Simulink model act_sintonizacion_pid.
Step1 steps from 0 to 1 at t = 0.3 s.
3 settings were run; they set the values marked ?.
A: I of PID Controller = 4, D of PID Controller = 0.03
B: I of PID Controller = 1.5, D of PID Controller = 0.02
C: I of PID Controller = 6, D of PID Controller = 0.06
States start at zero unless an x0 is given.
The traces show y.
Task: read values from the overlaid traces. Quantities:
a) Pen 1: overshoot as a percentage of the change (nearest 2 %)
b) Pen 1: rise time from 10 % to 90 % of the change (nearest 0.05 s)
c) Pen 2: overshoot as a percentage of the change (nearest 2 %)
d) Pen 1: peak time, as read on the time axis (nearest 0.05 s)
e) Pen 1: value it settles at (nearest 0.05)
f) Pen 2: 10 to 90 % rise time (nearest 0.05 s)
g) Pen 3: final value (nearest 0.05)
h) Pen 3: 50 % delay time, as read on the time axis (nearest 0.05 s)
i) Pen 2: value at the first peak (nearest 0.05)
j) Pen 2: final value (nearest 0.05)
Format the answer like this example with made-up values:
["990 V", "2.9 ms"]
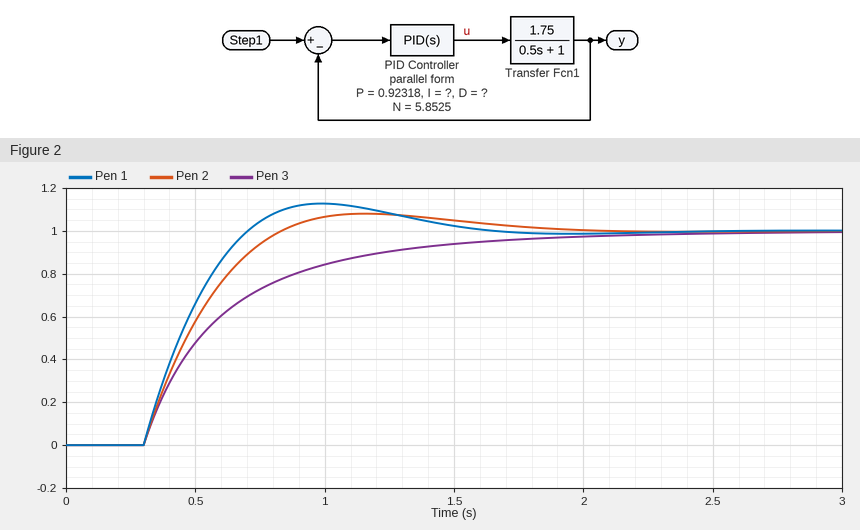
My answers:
["12 %", "0.30 s", "8 %", "1.00 s", "1.00", "0.40 s", "1.00", "0.50 s", "1.10", "1.00"]
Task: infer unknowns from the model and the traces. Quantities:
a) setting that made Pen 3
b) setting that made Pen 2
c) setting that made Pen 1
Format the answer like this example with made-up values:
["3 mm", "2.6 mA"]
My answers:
["B", "A", "C"]
